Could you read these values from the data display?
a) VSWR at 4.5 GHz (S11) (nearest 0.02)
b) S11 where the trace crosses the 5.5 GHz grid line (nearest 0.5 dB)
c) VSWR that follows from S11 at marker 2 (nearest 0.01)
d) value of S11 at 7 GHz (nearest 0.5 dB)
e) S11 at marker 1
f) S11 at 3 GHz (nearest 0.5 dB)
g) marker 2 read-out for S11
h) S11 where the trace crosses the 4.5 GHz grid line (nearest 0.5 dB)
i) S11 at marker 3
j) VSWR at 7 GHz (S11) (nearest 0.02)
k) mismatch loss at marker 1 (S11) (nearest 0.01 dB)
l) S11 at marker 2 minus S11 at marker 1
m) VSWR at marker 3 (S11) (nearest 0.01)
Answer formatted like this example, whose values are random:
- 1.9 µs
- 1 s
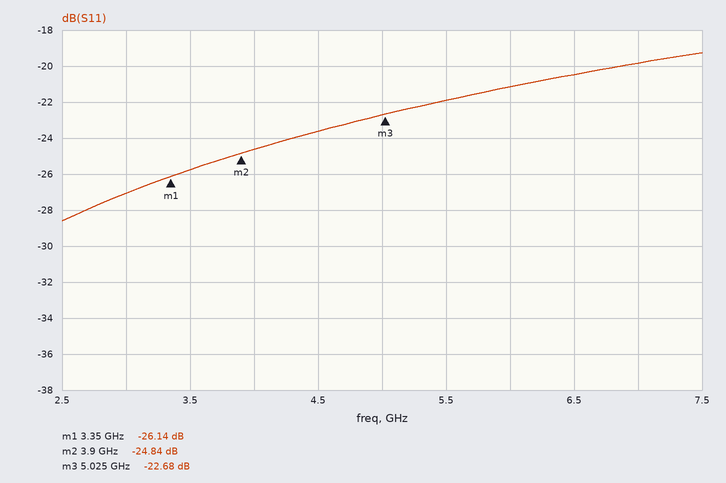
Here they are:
- 1.14
- -22.0 dB
- 1.12
- -20.0 dB
- -26.14 dB
- -27.0 dB
- -24.84 dB
- -23.5 dB
- -22.68 dB
- 1.22
- 0.01 dB
- 1.30 dB
- 1.16
